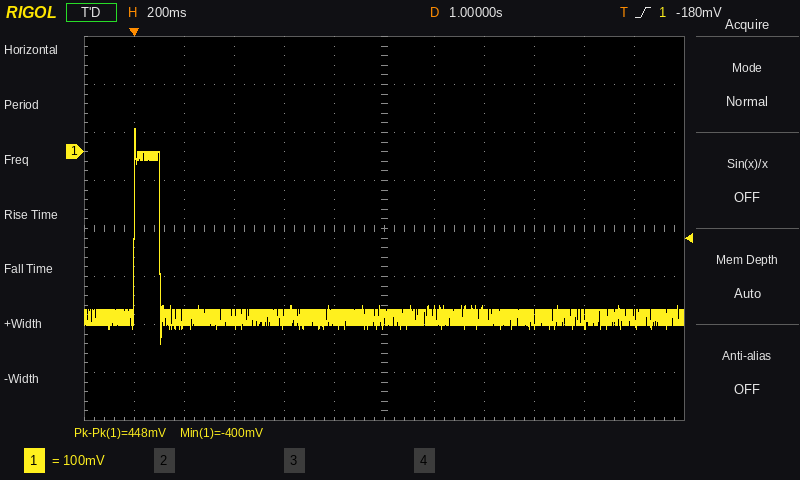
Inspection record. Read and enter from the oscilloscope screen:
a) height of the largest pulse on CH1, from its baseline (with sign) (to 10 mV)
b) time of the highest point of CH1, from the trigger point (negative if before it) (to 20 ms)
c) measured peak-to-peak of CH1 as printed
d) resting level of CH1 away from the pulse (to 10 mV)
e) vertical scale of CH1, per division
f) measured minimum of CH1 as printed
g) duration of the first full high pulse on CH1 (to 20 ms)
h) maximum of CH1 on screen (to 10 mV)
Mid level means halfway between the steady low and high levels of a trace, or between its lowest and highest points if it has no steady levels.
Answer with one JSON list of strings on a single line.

["+390 mV", "0 ms", "448 mV", "-340 mV", "100 mV", "-400 mV", "100 ms", "50 mV"]
